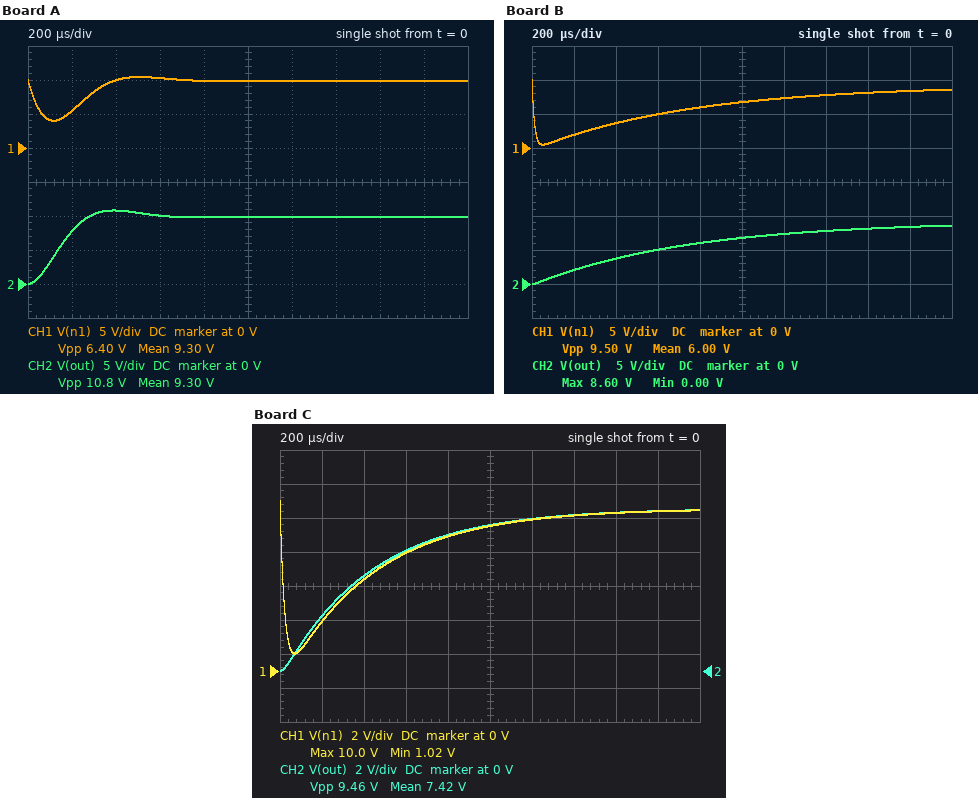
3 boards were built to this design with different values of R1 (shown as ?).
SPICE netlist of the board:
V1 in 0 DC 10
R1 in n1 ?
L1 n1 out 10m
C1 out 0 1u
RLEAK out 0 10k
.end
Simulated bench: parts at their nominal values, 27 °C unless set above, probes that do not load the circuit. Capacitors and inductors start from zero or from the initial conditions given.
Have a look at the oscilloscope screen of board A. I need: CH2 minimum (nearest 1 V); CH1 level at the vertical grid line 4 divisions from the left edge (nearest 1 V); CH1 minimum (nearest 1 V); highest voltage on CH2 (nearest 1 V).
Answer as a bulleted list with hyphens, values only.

- 0 V
- 10 V
- 4 V
- 11 V
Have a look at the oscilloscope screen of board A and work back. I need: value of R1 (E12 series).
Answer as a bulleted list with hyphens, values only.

- 120 Ω
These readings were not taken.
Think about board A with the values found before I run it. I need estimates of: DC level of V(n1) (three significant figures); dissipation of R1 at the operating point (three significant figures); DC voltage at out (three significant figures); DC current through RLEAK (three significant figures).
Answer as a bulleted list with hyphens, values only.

- 9.88 V
- 117 µW
- 9.88 V
- 988 µA
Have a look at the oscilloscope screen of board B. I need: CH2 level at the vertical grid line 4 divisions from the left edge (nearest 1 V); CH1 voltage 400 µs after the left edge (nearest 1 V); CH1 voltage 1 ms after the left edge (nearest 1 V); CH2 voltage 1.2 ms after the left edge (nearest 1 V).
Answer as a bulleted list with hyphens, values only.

- 6 V
- 4 V
- 7 V
- 7 V
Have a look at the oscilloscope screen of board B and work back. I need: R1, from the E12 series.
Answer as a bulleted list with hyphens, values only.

- 820 Ω
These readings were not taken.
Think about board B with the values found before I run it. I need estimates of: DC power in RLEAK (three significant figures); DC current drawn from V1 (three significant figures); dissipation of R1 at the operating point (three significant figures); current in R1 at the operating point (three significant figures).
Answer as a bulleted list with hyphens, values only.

- 8.54 mW
- 924 µA
- 700 µW
- 924 µA
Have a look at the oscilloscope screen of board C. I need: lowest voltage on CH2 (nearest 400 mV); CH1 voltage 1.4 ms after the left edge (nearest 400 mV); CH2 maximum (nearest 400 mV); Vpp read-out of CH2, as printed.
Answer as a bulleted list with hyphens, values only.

- 0 V
- 9.2 V
- 9.6 V
- 9.46 V
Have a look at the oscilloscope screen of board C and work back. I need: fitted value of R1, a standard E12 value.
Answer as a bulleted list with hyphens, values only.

- 470 Ω
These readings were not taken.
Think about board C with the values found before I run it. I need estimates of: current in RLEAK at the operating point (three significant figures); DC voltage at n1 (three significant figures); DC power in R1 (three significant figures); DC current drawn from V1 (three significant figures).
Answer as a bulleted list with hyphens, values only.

- 955 µA
- 9.55 V
- 429 µW
- 955 µA
